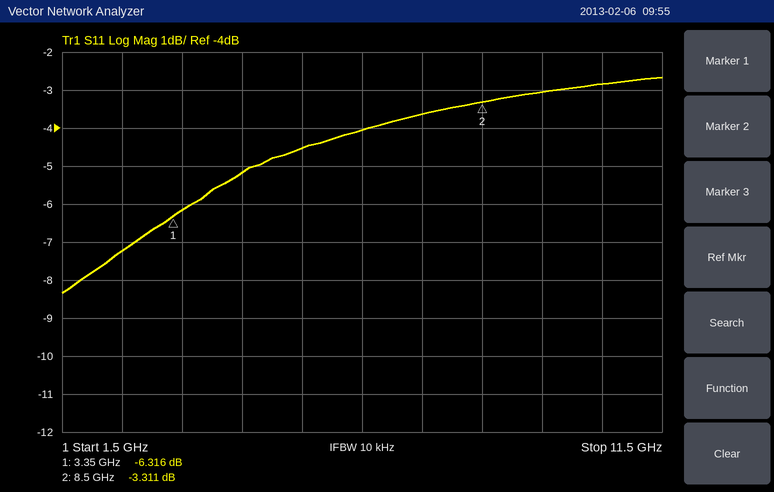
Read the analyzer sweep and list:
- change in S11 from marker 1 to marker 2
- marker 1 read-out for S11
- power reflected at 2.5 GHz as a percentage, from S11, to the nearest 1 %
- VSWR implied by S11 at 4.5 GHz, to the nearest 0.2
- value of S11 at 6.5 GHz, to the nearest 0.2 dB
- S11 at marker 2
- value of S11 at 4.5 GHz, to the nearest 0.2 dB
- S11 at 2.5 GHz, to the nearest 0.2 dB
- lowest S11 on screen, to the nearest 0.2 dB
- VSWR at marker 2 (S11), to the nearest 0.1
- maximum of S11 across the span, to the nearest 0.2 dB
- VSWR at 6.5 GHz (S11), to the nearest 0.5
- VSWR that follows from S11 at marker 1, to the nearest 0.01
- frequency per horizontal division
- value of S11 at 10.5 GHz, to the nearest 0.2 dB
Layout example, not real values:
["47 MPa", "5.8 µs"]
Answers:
["3.005 dB", "-6.316 dB", "19 %", "3.4", "-4.0 dB", "-3.311 dB", "-5.2 dB", "-7.2 dB", "-8.4 dB", "5.3", "-2.6 dB", "4.5", "2.87", "1 GHz", "-2.8 dB"]
